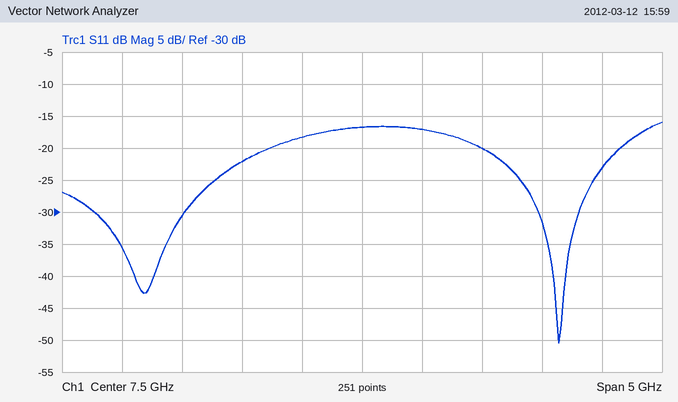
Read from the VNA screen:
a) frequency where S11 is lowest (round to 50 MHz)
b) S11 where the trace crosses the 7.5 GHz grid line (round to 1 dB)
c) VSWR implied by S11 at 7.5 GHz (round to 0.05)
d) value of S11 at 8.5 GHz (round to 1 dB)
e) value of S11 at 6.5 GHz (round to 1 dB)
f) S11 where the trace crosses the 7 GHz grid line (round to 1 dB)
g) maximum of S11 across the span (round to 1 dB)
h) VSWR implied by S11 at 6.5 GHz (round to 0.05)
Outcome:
9.15 GHz
-17 dB
1.35
-20 dB
-22 dB
-18 dB
-16 dB
1.15
